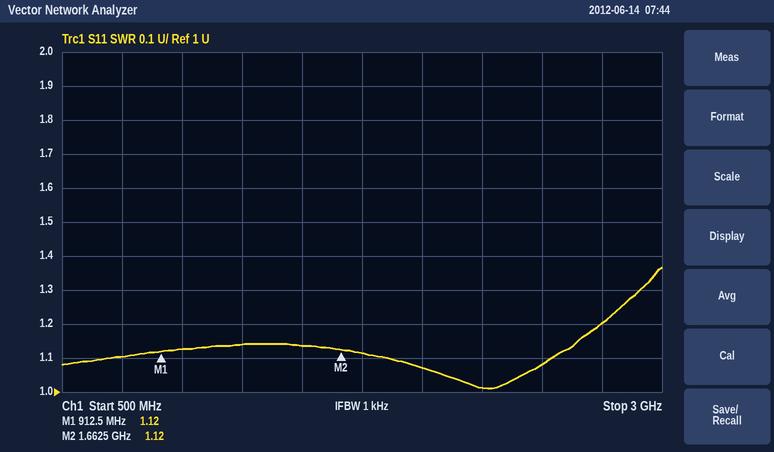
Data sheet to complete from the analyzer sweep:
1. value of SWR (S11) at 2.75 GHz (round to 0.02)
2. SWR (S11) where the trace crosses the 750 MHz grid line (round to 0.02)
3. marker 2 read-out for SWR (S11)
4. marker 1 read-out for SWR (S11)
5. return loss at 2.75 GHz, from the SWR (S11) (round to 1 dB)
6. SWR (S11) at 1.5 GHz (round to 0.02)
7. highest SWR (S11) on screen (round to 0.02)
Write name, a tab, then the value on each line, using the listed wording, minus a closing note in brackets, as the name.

value of SWR (S11) at 2.75 GHz	1.20
SWR (S11) where the trace crosses the 750 MHz grid line	1.10
marker 2 read-out for SWR	1.12
marker 1 read-out for SWR	1.12
return loss at 2.75 GHz, from the SWR (S11)	21 dB
SWR (S11) at 1.5 GHz	1.14
highest SWR (S11) on screen	1.36
